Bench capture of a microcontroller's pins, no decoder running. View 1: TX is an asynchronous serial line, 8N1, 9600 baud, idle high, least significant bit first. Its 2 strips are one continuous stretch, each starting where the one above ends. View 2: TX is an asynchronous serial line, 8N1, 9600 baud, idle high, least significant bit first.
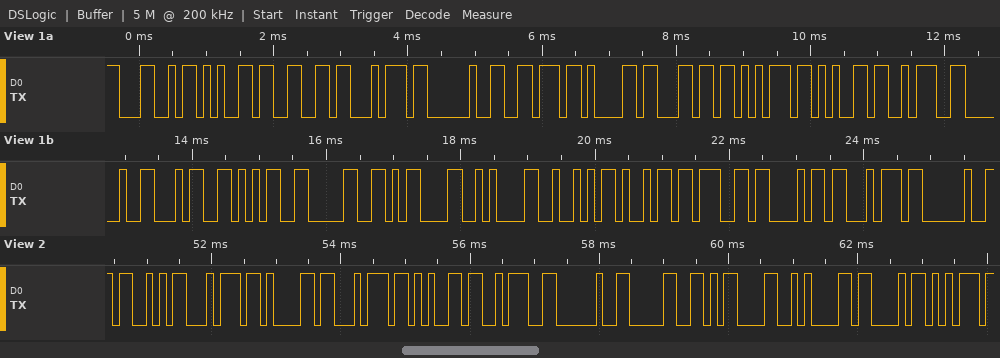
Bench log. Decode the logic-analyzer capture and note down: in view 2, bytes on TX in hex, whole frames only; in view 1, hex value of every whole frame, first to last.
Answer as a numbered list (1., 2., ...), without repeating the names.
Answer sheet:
1. 53 74 61 74 65 3A 20 30 0D 0A 43 75
2. 0x4C 0x65 0x66 0x74 0x20 0x76 0x61 0x6C 0x75 0x65 0x3A 0x20 0x34 0x35 0x30 0x0D 0x0A 0x52 0x69 0x67 0x68 0x74 0x20
